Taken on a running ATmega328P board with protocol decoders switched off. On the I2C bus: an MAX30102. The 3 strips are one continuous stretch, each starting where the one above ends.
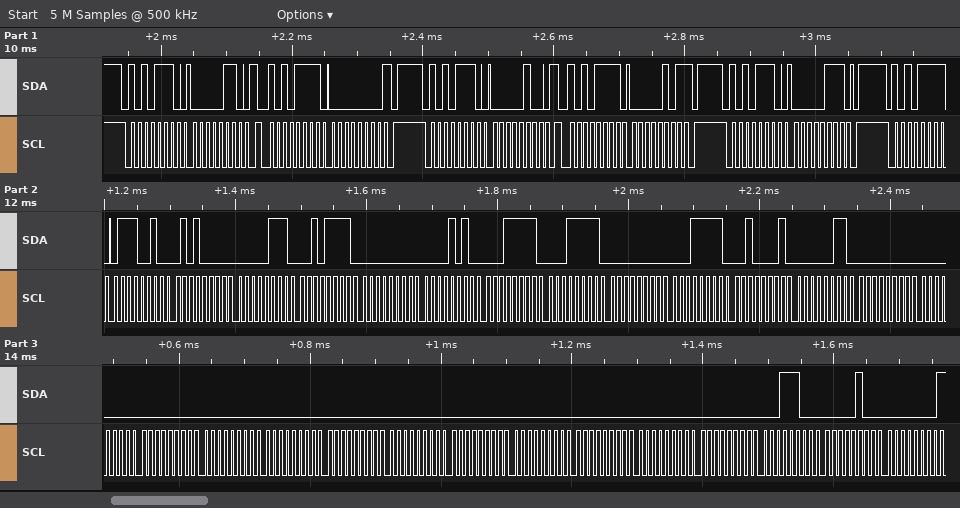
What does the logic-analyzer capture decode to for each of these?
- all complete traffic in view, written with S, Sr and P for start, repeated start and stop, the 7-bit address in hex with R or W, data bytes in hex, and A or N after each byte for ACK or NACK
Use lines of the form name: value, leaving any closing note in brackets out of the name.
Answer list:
all complete traffic in view, written with S, Sr and P for start, repeated start and stop, the 7-bit address in hex with R or W, data bytes in hex, and A or N after each byte for ACK or NACK: S 57W A 06 A Sr 57R A 00 N P S 57W A 04 A Sr 57R A 05 N P S 57W A 07 A P S 57R A 72 A 50 A 07 A 2F A 00 A 0A A 1F A 1F A 00 A 1F A 21 A 03 A 00 A 00 A 00 A 00 A 00 A 00 A 00 A 00 A 00 A 00 A 00 A 00 A 1C A 04 A 00 N
